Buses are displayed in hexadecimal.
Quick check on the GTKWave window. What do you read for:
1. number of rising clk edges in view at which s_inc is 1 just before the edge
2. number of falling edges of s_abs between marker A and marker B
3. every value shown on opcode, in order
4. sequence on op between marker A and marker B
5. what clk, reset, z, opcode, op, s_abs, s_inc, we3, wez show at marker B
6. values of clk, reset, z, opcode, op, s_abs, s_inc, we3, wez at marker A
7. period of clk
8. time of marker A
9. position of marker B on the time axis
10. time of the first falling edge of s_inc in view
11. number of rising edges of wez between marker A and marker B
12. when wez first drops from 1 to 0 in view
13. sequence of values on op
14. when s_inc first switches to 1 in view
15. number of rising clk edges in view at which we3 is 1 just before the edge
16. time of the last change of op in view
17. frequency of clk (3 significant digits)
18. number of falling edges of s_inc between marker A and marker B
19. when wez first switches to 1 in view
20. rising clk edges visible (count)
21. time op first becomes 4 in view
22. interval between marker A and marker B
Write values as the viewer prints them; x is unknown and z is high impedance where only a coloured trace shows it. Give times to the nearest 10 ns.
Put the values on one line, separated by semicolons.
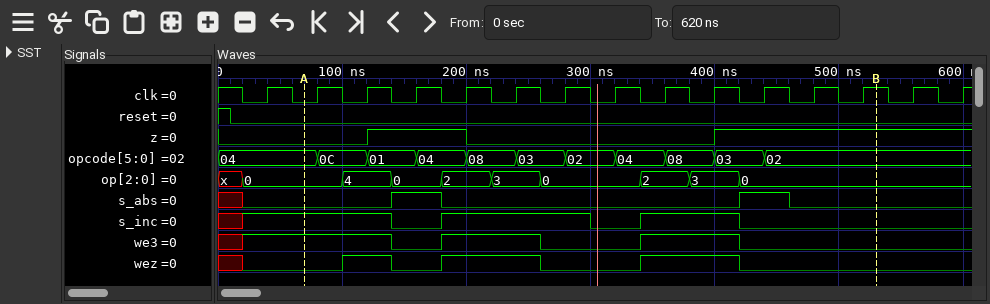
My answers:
8; 2; 04, 0C, 01, 04, 08, 03, 02, 04, 08, 03, 02; 0, 4, 0, 2, 3, 0, 2, 3, 0; clk=1, reset=0, z=1, opcode=02, op=0, s_abs=0, s_inc=0, we3=0, wez=0; clk=0, reset=0, z=0, opcode=04, op=0, s_abs=0, s_inc=1, we3=1, wez=0; 40 ns; 70 ns; 530 ns; 140 ns; 3; 140 ns; x, 0, 4, 0, 2, 3, 0, 2, 3, 0; 20 ns; 7; 420 ns; 25.0 MHz; 3; 100 ns; 15; 100 ns; 460 ns
